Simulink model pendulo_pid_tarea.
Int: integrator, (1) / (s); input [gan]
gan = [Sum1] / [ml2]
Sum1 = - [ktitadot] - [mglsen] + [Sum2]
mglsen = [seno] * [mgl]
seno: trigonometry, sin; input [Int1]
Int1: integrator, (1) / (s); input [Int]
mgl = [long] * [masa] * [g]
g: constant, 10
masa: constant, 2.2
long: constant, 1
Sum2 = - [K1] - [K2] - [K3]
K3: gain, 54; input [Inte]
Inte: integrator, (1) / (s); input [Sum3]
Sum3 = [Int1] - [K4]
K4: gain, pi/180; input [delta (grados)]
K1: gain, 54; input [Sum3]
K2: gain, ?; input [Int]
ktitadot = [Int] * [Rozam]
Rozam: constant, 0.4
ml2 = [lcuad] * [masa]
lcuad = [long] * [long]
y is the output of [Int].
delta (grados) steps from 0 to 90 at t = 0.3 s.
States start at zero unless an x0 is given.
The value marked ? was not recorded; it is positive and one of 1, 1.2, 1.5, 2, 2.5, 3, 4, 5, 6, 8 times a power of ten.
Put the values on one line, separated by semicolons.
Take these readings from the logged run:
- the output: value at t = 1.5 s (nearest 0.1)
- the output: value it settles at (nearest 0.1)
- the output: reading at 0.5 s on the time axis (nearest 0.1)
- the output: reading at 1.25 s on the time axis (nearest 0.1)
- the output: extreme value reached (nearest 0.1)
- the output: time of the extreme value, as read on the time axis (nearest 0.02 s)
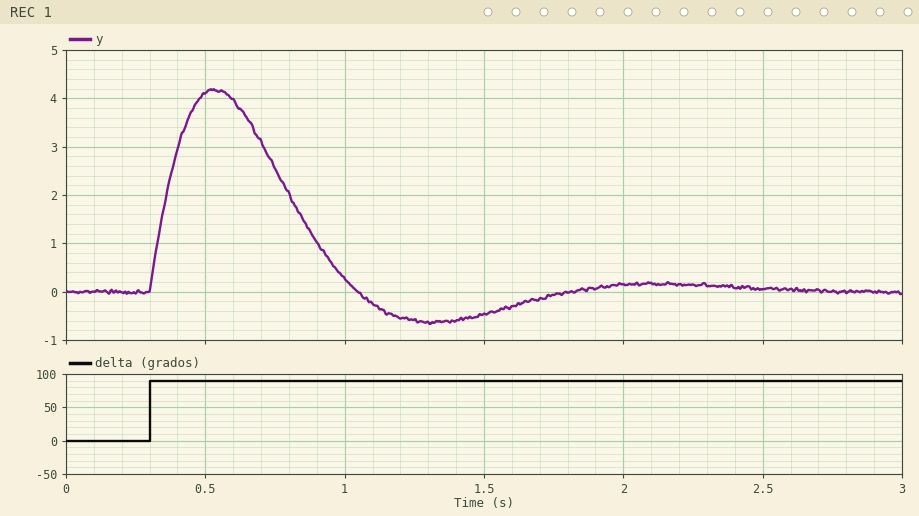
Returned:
-0.5; 0.0; 4.1; -0.6; 4.2; 0.54 s
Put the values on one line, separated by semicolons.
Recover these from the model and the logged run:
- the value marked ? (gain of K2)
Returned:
12
